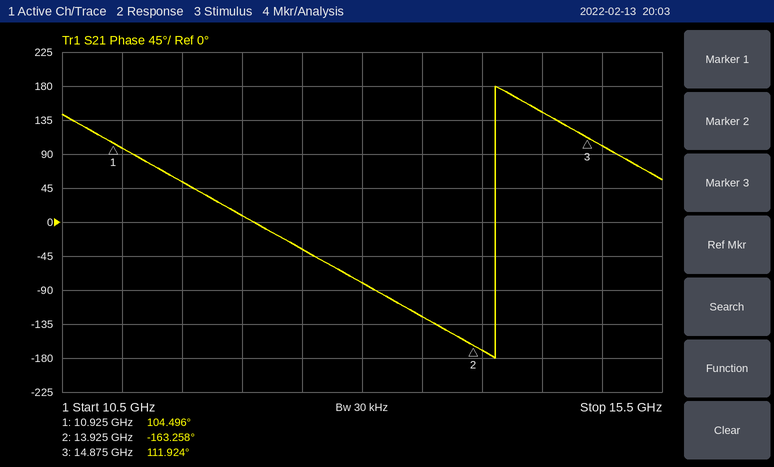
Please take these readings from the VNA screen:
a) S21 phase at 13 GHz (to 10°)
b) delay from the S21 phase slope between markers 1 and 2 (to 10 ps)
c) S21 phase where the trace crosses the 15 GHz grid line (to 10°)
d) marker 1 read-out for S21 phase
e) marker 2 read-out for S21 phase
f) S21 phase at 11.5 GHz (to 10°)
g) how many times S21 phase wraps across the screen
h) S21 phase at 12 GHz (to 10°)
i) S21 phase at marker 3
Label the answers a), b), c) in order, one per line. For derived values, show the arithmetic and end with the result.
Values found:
a) -80°
b) −(-163.258° − (104.496°))/(360° × 3 GHz) ≈ 248 ps, so 250 ps to the nearest 10 ps
c) 100°
d) 104.496°
e) -163.258°
f) 50°
g) 1
h) 10°
i) 111.924°
